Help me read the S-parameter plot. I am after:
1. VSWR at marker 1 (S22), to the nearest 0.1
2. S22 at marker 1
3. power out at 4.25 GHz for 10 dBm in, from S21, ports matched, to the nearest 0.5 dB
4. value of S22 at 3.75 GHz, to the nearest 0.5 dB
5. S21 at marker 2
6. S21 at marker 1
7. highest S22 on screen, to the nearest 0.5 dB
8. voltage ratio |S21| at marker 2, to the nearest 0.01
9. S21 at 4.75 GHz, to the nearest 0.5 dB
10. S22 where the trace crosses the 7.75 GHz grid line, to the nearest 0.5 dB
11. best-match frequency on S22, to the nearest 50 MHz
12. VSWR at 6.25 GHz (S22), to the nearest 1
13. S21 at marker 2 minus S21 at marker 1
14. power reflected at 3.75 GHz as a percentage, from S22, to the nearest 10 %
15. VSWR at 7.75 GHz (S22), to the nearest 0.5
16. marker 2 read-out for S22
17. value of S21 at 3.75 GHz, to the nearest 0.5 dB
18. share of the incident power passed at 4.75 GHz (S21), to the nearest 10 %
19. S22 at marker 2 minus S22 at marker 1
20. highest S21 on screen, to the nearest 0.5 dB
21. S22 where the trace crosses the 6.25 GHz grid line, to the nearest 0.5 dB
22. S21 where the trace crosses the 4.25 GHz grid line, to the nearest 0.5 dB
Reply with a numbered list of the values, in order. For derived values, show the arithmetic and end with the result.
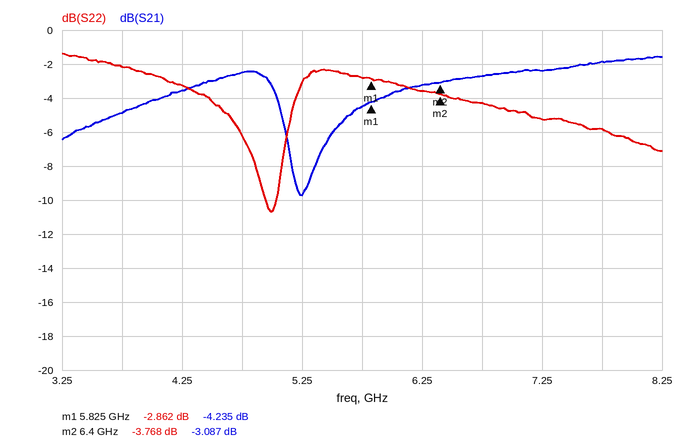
1. (1 + 0.7193)/(1 − 0.7193) ≈ 6.1
2. -2.862 dB
3. 10 dBm + (-3.5 dB) = 6.5 dBm
4. -2.0 dB
5. -3.087 dB
6. -4.235 dB
7. -1.5 dB
8. 10^(-3.087/20) ≈ 0.70
9. -2.5 dB
10. -6.0 dB
11. 5.00 GHz
12. |Γ| = 10^(-3.5/20) = 0.6683; VSWR = (1 + 0.6683)/(1 − 0.6683) ≈ 5
13. -3.087 − (-4.235) = 1.148 dB
14. 10^(-2/10) ≈ 63.1 %, so 60 % to the nearest 10 %
15. |Γ| = 10^(-6/20) = 0.5012; VSWR = (1 + 0.5012)/(1 − 0.5012) ≈ 3.0
16. -3.768 dB
17. -5.0 dB
18. 10^(-2.5/10) ≈ 56.2 %, so 60 % to the nearest 10 %
19. -3.768 − (-2.862) = -0.906 dB
20. -1.5 dB
21. -3.5 dB
22. -3.5 dB
